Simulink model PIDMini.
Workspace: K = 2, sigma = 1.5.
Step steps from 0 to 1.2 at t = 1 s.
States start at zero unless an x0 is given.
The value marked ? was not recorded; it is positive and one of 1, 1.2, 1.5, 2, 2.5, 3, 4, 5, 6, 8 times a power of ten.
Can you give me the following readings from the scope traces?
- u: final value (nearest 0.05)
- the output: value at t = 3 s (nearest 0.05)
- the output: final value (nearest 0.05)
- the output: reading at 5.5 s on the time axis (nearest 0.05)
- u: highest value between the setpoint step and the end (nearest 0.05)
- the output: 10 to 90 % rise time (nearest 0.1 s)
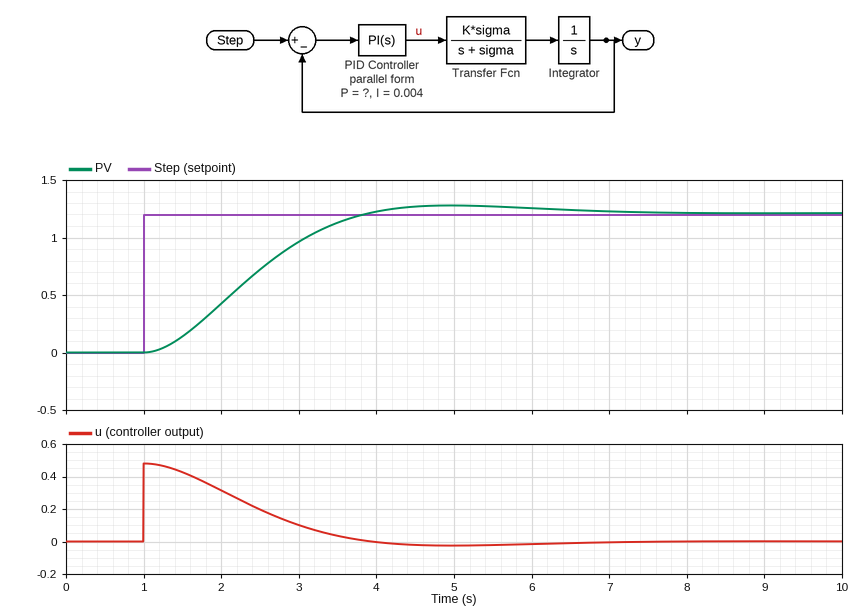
0.00
0.95
1.20
1.25
0.50
1.9 s
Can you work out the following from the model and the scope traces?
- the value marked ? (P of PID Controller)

0.4
